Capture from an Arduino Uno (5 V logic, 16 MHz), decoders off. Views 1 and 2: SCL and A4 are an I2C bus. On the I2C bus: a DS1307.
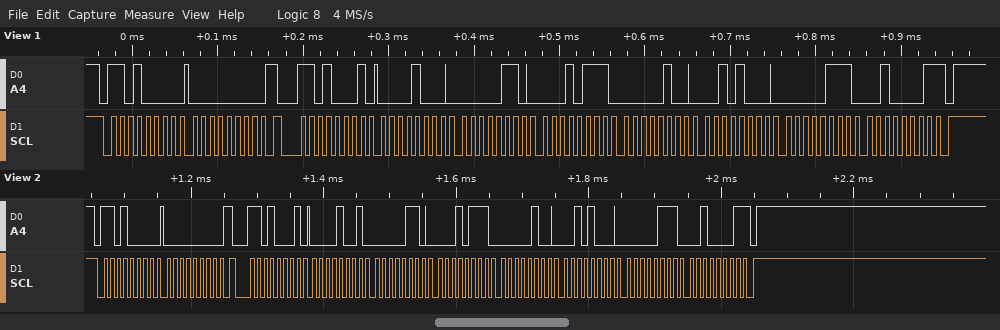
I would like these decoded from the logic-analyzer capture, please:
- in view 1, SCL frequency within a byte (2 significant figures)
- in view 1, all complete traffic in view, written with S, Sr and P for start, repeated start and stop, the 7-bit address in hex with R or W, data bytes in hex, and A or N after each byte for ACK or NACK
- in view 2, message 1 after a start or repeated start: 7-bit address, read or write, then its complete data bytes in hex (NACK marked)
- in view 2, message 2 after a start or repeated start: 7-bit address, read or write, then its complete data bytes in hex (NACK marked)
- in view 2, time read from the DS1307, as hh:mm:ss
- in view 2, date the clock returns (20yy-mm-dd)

100 kHz
S 68W A 00 A Sr 68R A 08 A 06 A 17 A 04 A 28 A 07 A 21 N P
0x68 write: 00
0x68 read: 09 06 17 04 28 07 21 NACK
17:06:09
2021-07-28
